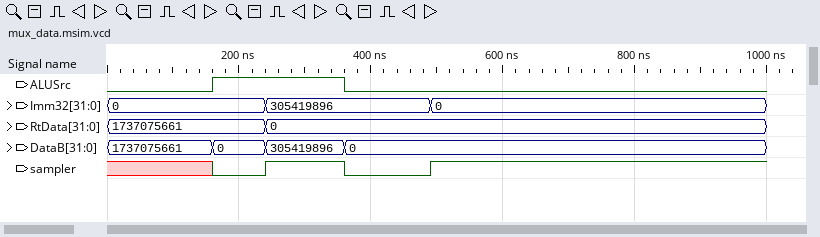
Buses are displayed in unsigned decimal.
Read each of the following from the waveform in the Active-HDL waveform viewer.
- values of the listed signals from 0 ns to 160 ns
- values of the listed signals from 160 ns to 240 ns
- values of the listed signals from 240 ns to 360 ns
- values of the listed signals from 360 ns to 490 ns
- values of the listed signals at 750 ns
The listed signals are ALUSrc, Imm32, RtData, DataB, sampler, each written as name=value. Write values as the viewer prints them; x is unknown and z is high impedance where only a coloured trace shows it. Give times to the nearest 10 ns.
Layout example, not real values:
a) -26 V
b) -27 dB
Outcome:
a) ALUSrc=0, Imm32=0, RtData=1737075661, DataB=1737075661, sampler=x
b) ALUSrc=1, Imm32=0, RtData=1737075661, DataB=0, sampler=0
c) ALUSrc=1, Imm32=305419896, RtData=0, DataB=305419896, sampler=1
d) ALUSrc=0, Imm32=305419896, RtData=0, DataB=0, sampler=0
e) ALUSrc=0, Imm32=0, RtData=0, DataB=0, sampler=1
